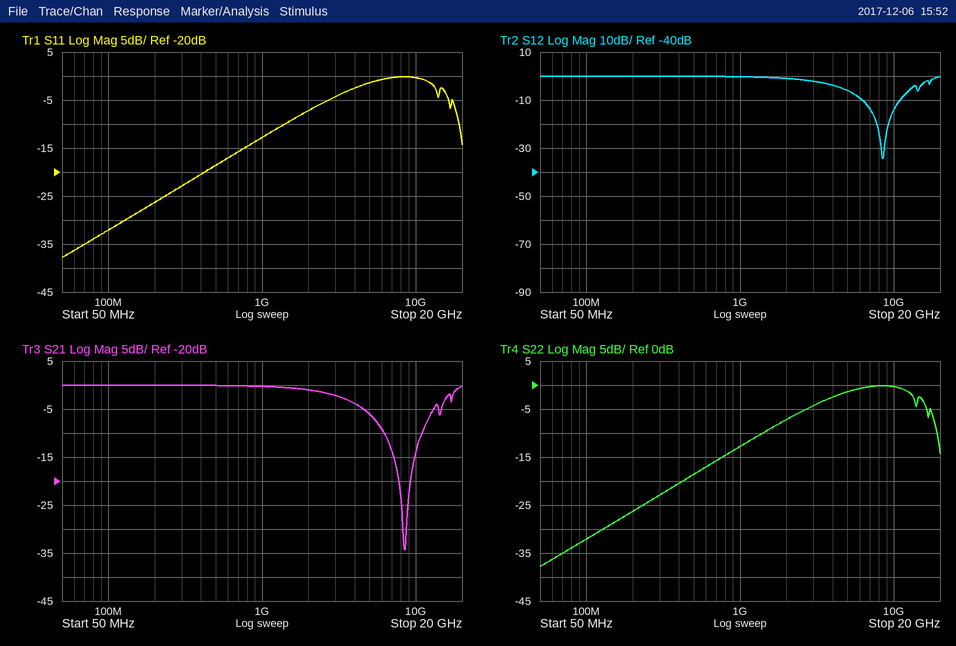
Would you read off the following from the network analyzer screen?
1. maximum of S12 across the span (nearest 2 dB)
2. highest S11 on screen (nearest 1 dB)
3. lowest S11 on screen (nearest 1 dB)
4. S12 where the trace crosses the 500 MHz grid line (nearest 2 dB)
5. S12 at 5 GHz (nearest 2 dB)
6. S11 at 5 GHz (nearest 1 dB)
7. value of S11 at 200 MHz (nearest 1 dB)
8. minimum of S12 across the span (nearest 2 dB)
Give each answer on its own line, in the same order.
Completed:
0 dB
0 dB
-38 dB
0 dB
-6 dB
-1 dB
-26 dB
-34 dB
